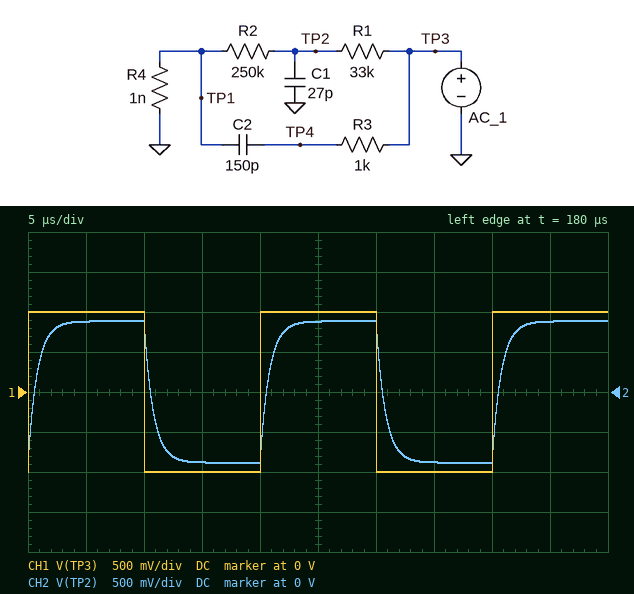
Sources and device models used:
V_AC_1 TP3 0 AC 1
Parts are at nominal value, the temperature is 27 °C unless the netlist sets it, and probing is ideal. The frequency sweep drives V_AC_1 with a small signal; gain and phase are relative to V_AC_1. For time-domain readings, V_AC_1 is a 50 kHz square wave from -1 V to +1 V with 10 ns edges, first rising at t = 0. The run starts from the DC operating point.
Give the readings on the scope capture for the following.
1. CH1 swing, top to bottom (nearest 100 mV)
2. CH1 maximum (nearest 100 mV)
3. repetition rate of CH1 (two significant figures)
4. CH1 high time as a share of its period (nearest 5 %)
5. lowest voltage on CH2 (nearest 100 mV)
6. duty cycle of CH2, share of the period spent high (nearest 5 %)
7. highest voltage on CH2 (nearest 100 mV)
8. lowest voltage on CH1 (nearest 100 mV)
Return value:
2.0 V
1.0 V
50 kHz
50 %
-900 mV
50 %
900 mV
-1.0 V
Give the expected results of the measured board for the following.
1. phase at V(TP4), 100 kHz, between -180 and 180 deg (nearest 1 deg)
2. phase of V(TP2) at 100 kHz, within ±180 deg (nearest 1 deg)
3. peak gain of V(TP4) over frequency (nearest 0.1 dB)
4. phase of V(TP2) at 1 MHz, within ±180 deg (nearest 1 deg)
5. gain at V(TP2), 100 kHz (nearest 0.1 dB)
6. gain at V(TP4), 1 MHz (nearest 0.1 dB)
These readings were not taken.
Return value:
-5 deg
-26 deg
0 dB
-79 deg
-2.0 dB
-2.8 dB
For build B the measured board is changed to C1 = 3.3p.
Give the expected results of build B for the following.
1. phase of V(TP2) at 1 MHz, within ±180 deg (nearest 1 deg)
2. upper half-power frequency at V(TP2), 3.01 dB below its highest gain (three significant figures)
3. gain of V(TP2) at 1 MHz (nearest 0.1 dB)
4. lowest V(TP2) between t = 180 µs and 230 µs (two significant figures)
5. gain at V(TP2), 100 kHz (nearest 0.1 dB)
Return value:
-31 deg
1.65 MHz
-2.4 dB
-880 mV
-1.1 dB
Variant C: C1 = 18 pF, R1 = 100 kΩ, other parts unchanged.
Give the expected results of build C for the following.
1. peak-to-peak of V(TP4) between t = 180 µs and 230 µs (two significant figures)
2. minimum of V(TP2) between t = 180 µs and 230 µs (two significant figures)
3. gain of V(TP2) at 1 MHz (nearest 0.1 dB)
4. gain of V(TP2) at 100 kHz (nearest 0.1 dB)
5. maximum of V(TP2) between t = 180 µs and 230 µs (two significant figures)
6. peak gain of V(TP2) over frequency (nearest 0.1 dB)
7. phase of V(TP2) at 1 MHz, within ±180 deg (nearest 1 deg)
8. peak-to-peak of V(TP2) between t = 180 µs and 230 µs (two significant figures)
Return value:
2.0 V
-710 mV
-21.1 dB
-5.1 dB
710 mV
-2.9 dB
-83 deg
1.4 V
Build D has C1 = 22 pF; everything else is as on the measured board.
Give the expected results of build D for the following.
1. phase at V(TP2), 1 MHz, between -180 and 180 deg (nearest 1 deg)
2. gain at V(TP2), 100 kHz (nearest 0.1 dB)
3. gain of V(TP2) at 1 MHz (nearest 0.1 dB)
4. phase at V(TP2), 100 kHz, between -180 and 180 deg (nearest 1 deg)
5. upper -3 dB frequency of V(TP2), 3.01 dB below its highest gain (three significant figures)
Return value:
-76 deg
-1.7 dB
-13.4 dB
-22 deg
248 kHz
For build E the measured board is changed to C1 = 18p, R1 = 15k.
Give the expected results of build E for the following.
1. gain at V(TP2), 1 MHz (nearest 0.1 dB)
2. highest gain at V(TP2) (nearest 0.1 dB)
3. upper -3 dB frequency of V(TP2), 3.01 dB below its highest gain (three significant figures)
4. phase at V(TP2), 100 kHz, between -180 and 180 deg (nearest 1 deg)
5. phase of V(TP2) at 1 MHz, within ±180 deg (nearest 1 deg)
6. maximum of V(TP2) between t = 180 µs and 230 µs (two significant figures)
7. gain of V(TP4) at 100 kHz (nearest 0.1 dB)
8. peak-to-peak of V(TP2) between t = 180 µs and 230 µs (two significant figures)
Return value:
-6.0 dB
-0.5 dB
625 kHz
-9 deg
-58 deg
940 mV
0 dB
1.9 V
